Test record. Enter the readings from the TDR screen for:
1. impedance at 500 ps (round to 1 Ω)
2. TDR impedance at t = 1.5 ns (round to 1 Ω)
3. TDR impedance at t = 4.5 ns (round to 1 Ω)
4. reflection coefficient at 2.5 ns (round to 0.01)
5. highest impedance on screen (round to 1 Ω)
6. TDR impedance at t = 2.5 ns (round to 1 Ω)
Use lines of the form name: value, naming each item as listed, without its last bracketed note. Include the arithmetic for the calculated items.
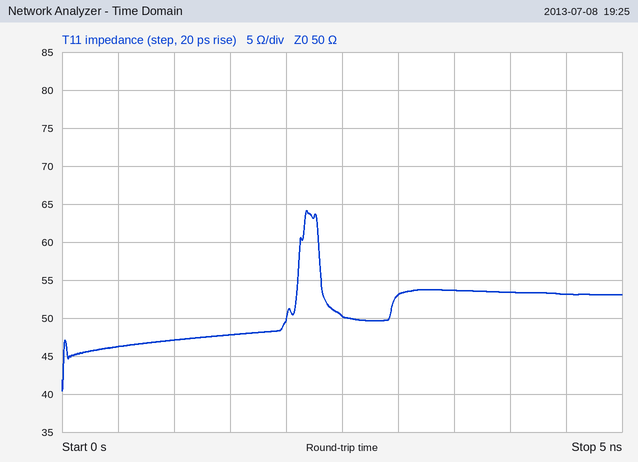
impedance at 500 ps: 46 Ω
TDR impedance at t = 1.5 ns: 48 Ω
TDR impedance at t = 4.5 ns: 53 Ω
reflection coefficient at 2.5 ns: (50 − 50)/(50 + 50) ≈ 0.00
highest impedance on screen: 64 Ω
TDR impedance at t = 2.5 ns: 50 Ω
